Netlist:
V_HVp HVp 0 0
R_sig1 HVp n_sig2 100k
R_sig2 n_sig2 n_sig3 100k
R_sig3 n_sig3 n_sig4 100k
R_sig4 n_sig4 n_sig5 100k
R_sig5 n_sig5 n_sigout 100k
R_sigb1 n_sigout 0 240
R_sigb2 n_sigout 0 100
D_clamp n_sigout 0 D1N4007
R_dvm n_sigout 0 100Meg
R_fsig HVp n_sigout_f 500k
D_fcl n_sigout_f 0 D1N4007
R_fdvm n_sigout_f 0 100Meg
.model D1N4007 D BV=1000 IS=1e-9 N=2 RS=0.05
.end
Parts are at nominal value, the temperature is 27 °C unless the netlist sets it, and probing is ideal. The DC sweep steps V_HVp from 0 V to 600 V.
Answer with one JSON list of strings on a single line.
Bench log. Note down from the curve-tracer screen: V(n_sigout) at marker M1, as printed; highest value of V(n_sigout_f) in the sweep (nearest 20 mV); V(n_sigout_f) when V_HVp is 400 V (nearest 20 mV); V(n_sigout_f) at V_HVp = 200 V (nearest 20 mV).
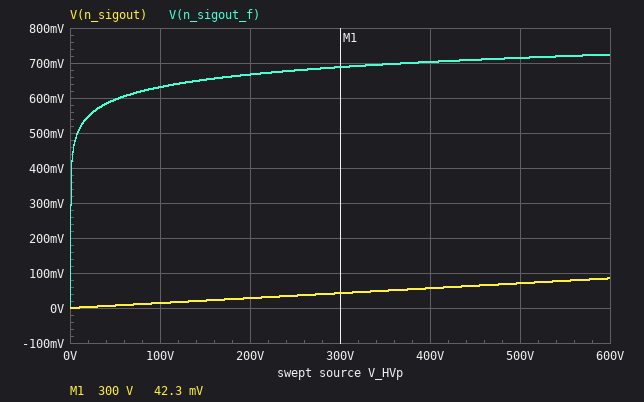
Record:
["42.3 mV", "720 mV", "700 mV", "660 mV"]
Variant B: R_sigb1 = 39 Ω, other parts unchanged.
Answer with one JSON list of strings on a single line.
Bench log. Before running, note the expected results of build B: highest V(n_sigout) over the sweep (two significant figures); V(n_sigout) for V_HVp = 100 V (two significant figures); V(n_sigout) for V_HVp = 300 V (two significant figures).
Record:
["34 mV", "5.6 mV", "17 mV"]
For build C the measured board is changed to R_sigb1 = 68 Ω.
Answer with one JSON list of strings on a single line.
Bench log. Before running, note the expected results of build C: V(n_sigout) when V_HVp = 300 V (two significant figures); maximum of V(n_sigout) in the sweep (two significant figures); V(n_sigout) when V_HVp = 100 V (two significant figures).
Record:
["24 mV", "49 mV", "8.1 mV"]
